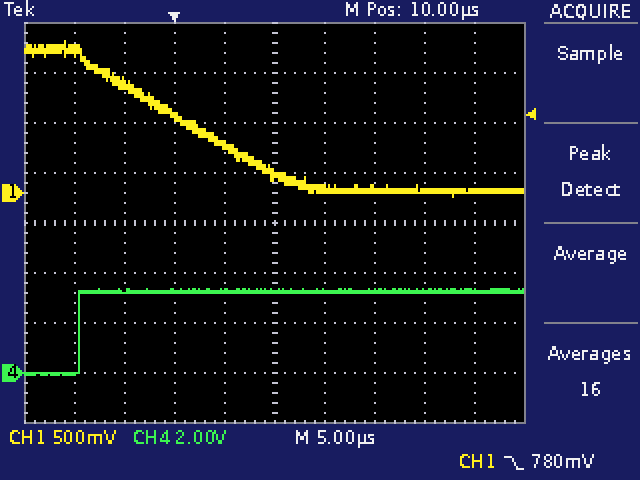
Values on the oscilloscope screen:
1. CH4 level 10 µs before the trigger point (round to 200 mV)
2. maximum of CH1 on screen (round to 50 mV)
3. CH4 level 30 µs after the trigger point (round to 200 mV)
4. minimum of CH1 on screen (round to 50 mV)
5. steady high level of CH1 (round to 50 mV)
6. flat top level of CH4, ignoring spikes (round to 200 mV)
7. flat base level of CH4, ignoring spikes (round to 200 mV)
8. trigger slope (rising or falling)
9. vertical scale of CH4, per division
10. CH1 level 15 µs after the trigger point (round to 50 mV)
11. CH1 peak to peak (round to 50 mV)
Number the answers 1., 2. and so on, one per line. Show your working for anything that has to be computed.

1. 0.0 V
2. 1.50 V
3. 3.2 V
4. -50 mV
5. 1.45 V
6. 3.2 V
7. 0.0 V
8. falling
9. 2 V
10. 50 mV
11. 1.50 V − (-50 mV) = 1.55 V
